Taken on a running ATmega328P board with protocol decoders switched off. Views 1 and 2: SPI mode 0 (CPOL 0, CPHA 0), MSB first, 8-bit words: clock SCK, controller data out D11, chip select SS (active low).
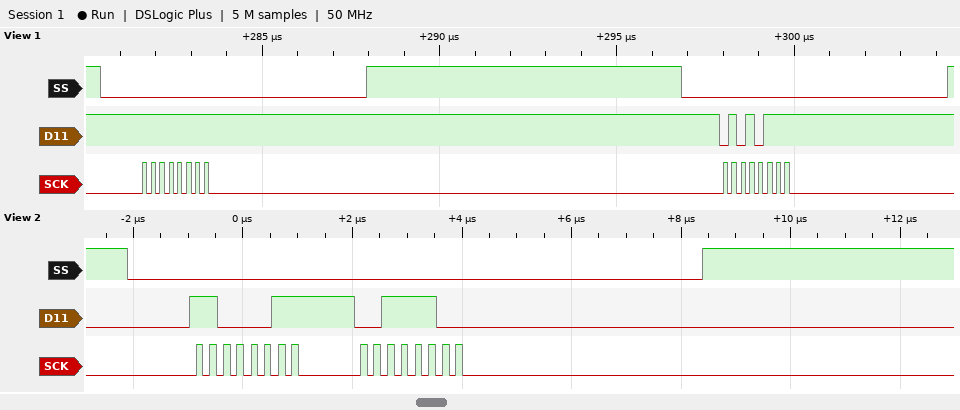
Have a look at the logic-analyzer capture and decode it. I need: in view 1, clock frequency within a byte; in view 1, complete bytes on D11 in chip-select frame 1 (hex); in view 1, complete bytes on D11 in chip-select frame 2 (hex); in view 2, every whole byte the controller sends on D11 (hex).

4 MHz
0xFF
0x57
C3 3C
